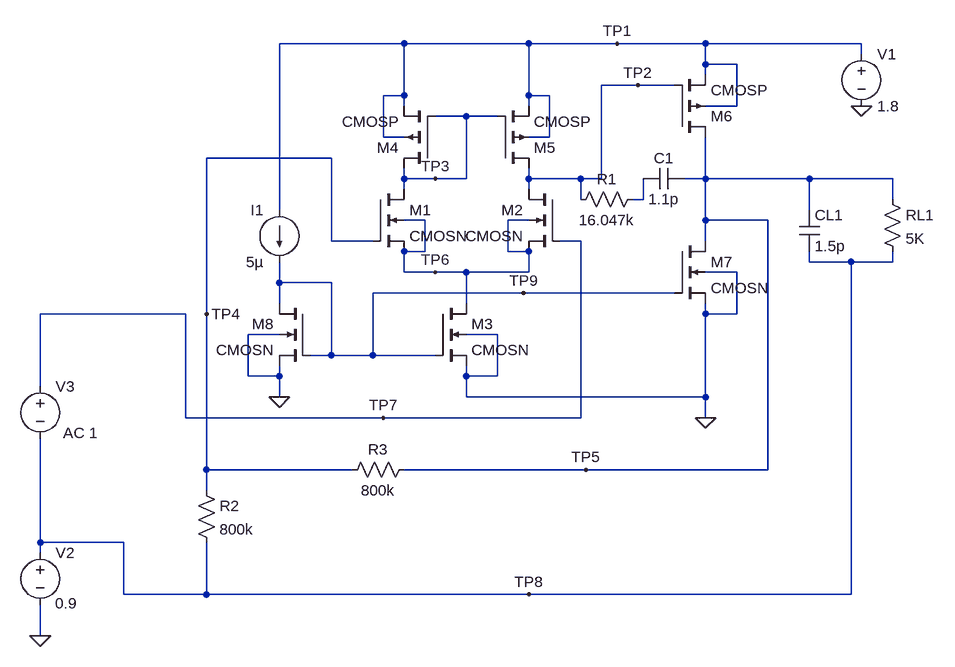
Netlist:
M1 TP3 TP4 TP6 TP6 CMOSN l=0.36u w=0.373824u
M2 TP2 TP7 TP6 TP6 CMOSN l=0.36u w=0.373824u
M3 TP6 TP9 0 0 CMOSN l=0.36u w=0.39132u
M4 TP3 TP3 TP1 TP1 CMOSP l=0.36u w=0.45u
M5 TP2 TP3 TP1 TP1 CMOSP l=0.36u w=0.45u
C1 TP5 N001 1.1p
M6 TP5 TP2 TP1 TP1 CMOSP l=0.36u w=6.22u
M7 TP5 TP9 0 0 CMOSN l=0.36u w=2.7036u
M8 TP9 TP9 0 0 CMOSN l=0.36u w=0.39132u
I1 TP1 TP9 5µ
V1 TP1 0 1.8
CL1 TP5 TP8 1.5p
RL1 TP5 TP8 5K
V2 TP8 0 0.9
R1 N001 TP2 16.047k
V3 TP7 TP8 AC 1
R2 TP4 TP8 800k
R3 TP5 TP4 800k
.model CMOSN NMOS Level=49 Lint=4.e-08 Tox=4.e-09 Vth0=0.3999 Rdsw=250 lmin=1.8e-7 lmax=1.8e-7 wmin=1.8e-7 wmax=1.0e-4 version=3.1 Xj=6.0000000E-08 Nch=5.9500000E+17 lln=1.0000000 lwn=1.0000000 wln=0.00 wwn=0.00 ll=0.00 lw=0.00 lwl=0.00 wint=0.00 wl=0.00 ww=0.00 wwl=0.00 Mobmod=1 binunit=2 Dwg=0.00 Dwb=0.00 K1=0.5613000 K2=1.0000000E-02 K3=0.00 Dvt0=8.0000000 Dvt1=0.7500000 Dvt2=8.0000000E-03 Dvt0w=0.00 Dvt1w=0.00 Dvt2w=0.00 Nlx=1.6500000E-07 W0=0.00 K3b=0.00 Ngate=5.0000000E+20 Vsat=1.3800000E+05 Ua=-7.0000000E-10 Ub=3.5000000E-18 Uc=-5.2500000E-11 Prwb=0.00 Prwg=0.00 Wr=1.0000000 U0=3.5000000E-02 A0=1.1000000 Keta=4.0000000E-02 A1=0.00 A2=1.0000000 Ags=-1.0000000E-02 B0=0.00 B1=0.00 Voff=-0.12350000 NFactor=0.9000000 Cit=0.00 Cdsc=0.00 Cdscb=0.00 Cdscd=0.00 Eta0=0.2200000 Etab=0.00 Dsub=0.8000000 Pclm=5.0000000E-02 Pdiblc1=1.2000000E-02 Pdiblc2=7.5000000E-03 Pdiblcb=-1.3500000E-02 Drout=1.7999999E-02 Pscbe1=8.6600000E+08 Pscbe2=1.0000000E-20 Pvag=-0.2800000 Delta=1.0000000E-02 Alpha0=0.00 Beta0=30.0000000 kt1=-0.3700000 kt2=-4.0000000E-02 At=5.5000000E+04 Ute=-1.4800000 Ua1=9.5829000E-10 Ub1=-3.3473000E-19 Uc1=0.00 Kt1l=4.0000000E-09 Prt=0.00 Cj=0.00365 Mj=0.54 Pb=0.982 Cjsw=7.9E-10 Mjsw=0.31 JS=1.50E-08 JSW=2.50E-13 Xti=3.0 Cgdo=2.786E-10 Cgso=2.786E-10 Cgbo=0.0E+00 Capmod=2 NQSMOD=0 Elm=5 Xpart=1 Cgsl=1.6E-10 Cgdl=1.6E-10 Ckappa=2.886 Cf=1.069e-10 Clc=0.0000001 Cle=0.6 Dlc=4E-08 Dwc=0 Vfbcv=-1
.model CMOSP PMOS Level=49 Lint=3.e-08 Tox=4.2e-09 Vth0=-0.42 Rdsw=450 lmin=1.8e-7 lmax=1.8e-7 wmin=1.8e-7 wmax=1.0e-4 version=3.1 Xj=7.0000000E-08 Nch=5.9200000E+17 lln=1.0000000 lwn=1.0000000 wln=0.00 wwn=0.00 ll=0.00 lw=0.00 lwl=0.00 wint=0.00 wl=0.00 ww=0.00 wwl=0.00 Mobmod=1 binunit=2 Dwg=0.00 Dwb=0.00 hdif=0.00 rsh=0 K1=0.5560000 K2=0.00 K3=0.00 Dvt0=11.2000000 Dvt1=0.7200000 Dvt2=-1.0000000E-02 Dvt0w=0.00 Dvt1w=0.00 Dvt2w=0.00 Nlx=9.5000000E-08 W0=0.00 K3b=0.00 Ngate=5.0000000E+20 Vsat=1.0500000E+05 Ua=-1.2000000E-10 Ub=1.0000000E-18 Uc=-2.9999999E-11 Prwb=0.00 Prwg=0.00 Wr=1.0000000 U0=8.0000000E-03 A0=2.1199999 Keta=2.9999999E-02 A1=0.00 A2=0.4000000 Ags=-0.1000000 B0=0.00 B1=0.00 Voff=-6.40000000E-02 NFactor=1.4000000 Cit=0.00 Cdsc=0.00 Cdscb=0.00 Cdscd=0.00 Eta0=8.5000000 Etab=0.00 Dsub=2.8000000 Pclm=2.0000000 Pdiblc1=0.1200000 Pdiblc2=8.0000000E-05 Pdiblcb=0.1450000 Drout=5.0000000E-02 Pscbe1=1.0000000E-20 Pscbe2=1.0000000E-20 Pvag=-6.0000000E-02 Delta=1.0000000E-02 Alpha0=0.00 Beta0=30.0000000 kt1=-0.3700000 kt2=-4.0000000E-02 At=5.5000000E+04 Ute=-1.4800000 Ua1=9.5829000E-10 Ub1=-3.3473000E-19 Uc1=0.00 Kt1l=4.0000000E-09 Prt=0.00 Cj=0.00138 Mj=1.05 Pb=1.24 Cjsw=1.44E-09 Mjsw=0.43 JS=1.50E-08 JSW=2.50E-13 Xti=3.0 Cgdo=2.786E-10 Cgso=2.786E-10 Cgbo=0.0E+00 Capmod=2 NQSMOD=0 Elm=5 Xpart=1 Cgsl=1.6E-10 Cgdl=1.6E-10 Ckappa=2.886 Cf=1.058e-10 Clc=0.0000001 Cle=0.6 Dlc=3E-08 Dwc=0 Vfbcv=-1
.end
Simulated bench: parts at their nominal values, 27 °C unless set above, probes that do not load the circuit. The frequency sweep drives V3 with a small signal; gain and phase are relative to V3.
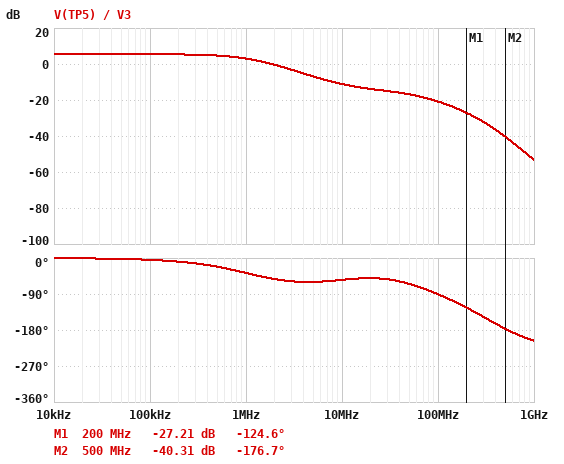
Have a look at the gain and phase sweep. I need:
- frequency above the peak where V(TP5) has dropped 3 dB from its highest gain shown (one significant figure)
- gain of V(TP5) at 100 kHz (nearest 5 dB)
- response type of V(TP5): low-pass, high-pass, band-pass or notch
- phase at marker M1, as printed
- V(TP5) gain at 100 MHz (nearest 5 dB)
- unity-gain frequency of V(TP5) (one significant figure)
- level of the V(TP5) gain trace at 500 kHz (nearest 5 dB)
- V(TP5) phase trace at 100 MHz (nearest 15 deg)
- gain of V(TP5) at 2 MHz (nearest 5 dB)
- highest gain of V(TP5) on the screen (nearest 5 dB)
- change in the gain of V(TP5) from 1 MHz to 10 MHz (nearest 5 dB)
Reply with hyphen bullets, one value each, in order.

- 1 MHz
- 5 dB
- low-pass
- -124.6 deg
- -20 dB
- 2 MHz
- 5 dB
- -90 deg
- 0 dB
- 5 dB
- -15 dB
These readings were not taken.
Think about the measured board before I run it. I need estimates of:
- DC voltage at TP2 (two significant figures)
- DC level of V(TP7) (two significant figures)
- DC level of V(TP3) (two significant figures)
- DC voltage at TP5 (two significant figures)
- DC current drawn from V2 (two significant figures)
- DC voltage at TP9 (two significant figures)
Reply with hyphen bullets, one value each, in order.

- 1.1 V
- 900 mV
- 1.1 V
- 900 mV
- 160 nA
- 680 mV
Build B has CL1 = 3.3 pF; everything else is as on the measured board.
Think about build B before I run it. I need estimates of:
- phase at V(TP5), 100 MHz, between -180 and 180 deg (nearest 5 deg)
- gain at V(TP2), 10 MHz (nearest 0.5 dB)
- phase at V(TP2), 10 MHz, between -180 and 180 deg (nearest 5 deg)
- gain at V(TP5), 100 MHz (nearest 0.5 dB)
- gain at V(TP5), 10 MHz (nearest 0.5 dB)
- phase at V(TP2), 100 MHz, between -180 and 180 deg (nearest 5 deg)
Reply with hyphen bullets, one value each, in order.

- -105 deg
- -8.5 dB
- 165 deg
- -27.0 dB
- -11.5 dB
- 160 deg
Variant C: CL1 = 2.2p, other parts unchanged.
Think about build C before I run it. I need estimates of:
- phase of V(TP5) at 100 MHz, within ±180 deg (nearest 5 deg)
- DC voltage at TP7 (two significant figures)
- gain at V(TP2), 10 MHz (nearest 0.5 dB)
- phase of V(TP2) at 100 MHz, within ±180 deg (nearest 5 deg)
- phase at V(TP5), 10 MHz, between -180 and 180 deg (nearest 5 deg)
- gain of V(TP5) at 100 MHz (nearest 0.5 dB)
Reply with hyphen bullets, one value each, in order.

- -100 deg
- 900 mV
- -9.5 dB
- 160 deg
- -60 deg
- -23.5 dB
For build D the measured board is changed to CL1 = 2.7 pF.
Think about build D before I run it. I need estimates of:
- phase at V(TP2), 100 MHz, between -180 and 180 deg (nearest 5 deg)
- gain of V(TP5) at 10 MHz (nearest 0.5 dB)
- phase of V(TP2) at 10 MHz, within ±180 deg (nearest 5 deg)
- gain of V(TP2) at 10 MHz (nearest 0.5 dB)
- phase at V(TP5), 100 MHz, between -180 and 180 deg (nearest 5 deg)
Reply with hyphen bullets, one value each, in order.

- 160 deg
- -11.5 dB
- 165 deg
- -9.0 dB
- -105 deg
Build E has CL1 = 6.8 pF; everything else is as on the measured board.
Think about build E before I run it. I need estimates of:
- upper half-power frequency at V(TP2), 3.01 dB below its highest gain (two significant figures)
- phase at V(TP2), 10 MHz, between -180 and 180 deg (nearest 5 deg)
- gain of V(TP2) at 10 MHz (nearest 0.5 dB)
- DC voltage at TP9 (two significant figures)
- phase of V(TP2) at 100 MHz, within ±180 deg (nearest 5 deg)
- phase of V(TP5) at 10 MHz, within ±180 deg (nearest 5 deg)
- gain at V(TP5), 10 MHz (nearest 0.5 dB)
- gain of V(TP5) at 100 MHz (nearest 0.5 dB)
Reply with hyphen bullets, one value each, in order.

- 1.4 MHz
- 165 deg
- -6.5 dB
- 680 mV
- 155 deg
- -85 deg
- -13.0 dB
- -33.0 dB
